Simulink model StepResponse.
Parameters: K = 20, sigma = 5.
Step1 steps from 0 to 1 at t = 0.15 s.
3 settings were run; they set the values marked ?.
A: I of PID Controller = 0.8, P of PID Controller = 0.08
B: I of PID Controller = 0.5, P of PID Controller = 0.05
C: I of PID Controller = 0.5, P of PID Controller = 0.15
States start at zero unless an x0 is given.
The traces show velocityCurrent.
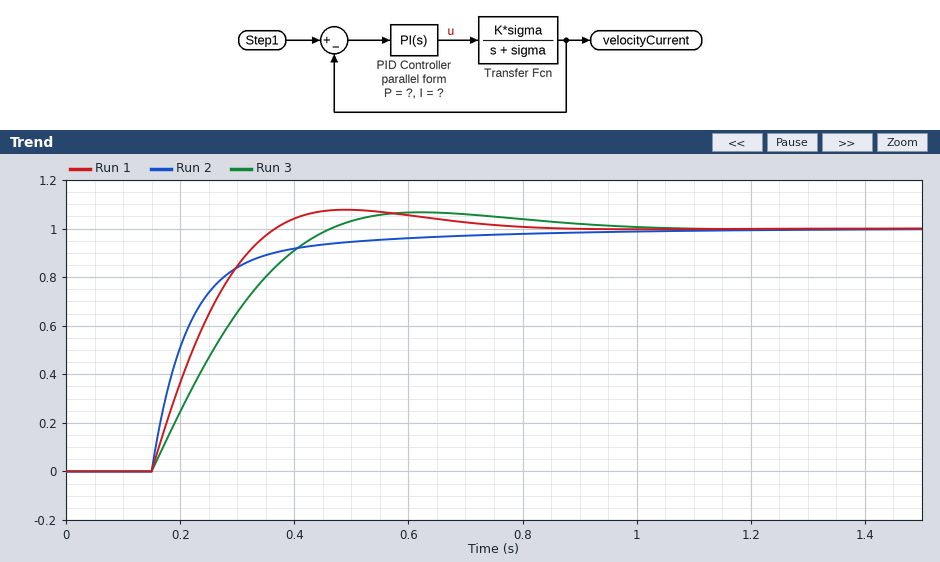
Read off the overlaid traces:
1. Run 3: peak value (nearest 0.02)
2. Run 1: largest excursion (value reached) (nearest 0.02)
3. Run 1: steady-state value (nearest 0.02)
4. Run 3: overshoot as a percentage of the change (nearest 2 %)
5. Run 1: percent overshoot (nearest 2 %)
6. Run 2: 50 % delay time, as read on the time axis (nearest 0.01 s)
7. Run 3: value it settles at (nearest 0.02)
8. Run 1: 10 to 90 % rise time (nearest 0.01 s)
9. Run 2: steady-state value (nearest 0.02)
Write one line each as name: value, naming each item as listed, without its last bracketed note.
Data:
Run 3: peak value: 1.06
Run 1: largest excursion (value reached): 1.08
Run 1: steady-state value: 1.00
Run 3: overshoot as a percentage of the change: 6 %
Run 1: percent overshoot: 8 %
Run 2: 50 % delay time, as read on the time axis: 0.20 s
Run 3: value it settles at: 1.00
Run 1: 10 to 90 % rise time: 0.16 s
Run 2: steady-state value: 1.00
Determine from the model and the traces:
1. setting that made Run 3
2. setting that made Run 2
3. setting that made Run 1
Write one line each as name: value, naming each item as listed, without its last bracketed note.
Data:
setting that made Run 3: B
setting that made Run 2: C
setting that made Run 1: A
